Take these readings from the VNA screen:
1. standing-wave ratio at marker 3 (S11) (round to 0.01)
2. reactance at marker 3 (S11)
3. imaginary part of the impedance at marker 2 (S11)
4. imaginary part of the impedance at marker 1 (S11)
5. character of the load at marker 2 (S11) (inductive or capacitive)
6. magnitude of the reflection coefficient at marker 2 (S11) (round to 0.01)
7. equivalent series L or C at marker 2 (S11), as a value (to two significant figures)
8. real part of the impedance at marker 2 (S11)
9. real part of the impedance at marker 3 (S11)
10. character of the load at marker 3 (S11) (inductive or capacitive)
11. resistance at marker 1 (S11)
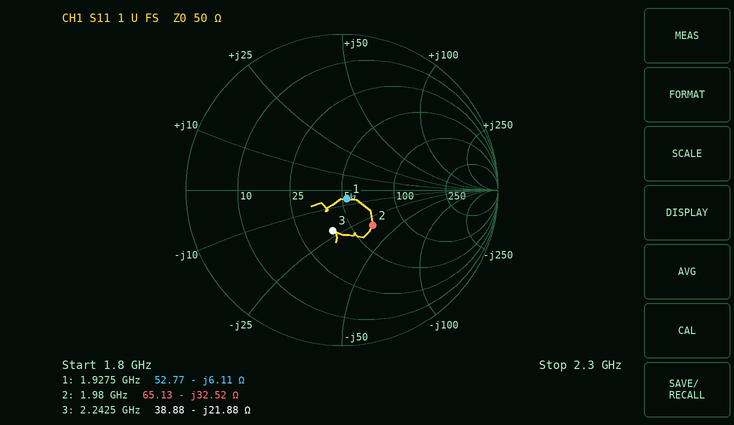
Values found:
1.73
-21.88 Ω
-32.52 Ω
-6.11 Ω
capacitive
0.30
2.5 pF
65.13 Ω
38.88 Ω
capacitive
52.77 Ω
